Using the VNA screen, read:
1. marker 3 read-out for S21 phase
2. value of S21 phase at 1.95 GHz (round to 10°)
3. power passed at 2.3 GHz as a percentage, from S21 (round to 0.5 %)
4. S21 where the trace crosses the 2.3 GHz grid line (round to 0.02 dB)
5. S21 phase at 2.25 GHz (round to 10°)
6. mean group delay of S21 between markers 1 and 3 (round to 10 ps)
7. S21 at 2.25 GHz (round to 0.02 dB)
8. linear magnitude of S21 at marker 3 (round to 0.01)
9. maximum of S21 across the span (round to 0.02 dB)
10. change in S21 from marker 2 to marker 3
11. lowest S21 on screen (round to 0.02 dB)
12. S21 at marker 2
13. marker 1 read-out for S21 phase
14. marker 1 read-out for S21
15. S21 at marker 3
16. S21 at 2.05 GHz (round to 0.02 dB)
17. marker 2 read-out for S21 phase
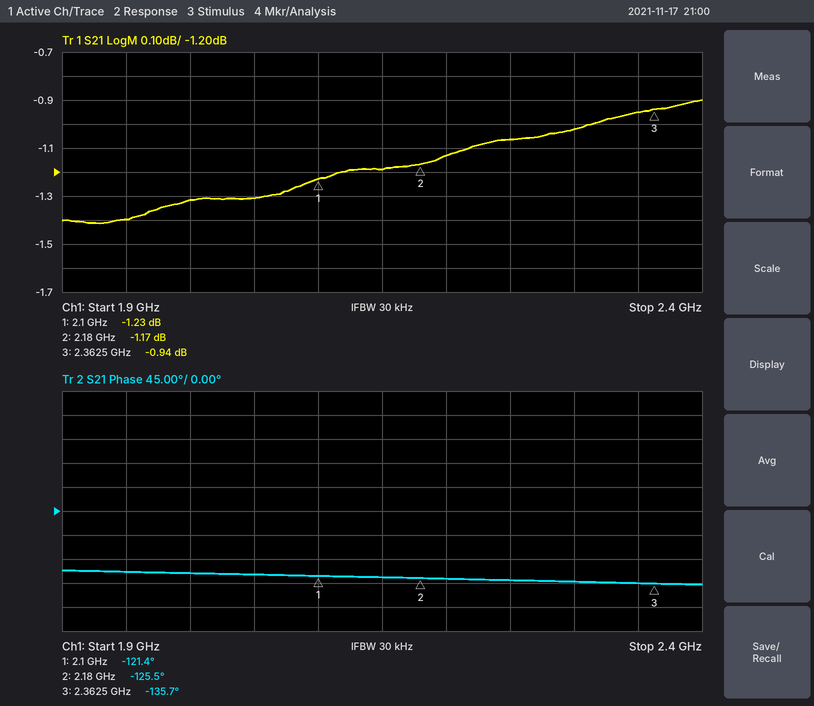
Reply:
-135.7°
-110°
79.0 %
-1.02 dB
-130°
150 ps
-1.06 dB
0.90
-0.90 dB
0.23 dB
-1.42 dB
-1.17 dB
-121.4°
-1.23 dB
-0.94 dB
-1.30 dB
-125.5°
